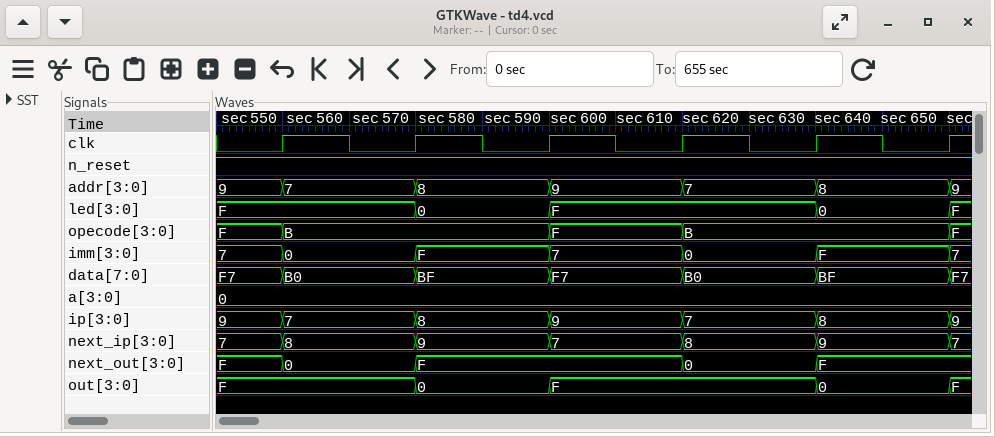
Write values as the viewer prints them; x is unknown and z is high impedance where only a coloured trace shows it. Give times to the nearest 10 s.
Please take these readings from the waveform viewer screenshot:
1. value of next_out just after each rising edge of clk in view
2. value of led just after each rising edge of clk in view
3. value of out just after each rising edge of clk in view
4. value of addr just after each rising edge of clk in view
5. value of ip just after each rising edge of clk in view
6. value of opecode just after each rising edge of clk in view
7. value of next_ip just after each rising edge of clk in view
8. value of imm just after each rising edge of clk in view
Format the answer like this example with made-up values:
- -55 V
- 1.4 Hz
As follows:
- 0, F, F, 0, F, F
- F, 0, F, F, 0, F
- F, 0, F, F, 0, F
- 7, 8, 9, 7, 8, 9
- 7, 8, 9, 7, 8, 9
- B, B, F, B, B, F
- 8, 9, 7, 8, 9, 7
- 0, F, 7, 0, F, 7
